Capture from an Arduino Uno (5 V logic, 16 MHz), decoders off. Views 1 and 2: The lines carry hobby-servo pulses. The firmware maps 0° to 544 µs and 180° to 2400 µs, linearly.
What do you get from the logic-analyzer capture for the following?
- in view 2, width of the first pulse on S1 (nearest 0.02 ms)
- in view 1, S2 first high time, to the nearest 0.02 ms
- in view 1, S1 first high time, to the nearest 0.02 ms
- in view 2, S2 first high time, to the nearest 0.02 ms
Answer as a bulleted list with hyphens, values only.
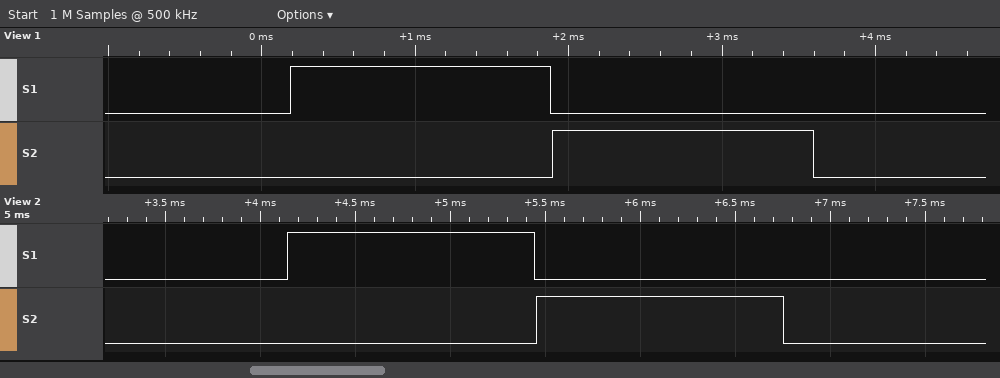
- 1.30 ms
- 1.70 ms
- 1.70 ms
- 1.30 ms
